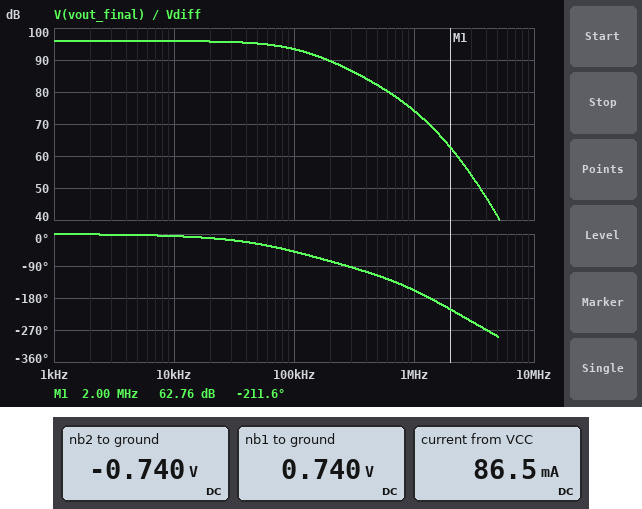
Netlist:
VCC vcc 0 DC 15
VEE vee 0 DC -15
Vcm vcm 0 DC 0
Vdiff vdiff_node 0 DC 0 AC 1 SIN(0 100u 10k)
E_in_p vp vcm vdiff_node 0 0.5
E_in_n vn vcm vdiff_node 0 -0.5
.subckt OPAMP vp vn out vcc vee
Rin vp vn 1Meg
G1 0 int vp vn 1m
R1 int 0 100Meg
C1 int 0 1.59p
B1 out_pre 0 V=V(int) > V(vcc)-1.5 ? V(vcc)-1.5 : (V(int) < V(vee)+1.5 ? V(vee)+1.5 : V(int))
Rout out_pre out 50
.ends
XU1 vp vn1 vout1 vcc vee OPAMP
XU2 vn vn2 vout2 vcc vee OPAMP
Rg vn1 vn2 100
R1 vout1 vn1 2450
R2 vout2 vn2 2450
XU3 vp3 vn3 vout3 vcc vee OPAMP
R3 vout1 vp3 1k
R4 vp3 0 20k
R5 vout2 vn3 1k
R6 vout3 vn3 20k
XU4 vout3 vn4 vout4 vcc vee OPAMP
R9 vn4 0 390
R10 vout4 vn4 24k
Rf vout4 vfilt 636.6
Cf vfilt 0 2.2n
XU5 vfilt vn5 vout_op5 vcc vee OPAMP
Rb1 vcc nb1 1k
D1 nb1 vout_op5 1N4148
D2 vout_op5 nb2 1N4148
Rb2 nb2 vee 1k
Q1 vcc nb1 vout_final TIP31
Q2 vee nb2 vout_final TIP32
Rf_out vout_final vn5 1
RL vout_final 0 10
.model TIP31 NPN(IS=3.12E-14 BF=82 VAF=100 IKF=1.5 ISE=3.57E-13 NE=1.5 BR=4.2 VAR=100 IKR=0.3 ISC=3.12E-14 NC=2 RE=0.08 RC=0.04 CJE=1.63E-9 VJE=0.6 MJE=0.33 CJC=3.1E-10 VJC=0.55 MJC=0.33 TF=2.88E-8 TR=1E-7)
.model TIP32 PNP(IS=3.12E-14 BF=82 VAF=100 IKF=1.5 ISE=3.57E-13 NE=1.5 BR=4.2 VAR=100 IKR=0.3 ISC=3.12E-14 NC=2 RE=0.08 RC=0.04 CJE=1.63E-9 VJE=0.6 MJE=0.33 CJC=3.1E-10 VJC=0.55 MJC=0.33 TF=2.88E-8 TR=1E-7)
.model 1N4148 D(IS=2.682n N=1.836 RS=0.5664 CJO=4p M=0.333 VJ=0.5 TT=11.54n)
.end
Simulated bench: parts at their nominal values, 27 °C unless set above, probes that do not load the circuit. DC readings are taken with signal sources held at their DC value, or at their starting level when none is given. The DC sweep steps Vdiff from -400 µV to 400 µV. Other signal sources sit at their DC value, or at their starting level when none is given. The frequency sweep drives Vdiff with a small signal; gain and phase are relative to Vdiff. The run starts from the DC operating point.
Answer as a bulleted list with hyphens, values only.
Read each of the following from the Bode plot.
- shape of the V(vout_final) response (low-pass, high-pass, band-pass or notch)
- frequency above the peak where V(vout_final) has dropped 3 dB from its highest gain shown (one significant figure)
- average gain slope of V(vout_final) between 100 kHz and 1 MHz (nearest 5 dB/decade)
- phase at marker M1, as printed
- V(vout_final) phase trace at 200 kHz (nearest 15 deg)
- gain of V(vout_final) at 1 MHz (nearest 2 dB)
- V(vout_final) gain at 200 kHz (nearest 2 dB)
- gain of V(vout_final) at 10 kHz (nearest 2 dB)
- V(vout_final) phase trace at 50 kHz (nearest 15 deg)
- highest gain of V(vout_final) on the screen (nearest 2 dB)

- low-pass
- 100 kHz
- -20 dB/decade
- -211.6 deg
- -75 deg
- 74 dB
- 90 dB
- 96 dB
- -30 deg
- 96 dB
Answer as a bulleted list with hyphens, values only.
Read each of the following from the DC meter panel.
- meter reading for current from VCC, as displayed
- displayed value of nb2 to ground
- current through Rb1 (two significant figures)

- 86.5 mA
- -0.740 V
- 14 mA
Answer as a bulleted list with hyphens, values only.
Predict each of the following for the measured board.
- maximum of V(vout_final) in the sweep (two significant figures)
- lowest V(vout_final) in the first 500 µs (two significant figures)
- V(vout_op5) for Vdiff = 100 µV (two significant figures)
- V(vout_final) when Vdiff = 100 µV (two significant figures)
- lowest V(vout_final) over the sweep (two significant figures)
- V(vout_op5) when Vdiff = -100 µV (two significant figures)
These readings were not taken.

- 5.6 V
- -5.6 V
- 12 V
- 5.6 V
- -5.6 V
- -12 V
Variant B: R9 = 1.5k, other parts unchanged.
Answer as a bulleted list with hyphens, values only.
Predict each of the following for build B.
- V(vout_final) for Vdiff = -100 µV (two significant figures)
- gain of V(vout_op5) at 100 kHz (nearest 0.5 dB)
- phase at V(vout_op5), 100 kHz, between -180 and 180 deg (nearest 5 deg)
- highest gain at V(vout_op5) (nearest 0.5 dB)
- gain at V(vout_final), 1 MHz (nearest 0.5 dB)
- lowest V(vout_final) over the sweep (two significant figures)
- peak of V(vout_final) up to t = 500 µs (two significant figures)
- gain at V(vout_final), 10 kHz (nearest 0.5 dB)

- -1.7 V
- 82.5 dB
- -45 deg
- 85.0 dB
- 64.5 dB
- -5.6 V
- 1.7 V
- 84.5 dB
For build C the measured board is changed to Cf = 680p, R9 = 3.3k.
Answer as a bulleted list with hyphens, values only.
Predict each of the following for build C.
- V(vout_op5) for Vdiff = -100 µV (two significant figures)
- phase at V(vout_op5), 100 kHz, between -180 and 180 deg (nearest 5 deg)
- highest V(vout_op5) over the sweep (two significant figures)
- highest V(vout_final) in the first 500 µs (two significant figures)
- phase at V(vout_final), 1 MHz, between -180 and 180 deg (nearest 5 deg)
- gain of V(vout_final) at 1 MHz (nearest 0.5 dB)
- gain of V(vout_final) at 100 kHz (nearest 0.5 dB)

- -850 mV
- -20 deg
- 3.4 V
- 830 mV
- -115 deg
- 68.0 dB
- 78.0 dB
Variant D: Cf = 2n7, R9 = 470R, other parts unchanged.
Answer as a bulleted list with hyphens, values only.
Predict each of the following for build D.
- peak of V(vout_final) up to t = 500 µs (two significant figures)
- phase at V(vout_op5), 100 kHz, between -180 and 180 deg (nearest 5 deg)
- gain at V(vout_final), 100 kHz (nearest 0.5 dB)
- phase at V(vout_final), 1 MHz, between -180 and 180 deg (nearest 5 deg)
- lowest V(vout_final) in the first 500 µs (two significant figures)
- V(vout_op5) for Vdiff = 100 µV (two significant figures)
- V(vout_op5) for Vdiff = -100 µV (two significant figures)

- 5.2 V
- -55 deg
- 91.0 dB
- -155 deg
- -5.2 V
- 5.4 V
- -5.4 V
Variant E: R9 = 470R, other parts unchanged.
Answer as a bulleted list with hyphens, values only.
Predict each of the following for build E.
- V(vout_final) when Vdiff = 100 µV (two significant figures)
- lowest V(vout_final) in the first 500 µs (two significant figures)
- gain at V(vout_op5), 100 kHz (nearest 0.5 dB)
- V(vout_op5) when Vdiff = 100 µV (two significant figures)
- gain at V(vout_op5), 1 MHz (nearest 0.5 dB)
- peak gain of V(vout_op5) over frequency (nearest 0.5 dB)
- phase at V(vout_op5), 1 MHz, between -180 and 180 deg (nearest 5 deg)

- 5.2 V
- -5.2 V
- 92.0 dB
- 5.4 V
- 73.5 dB
- 94.5 dB
- -150 deg
